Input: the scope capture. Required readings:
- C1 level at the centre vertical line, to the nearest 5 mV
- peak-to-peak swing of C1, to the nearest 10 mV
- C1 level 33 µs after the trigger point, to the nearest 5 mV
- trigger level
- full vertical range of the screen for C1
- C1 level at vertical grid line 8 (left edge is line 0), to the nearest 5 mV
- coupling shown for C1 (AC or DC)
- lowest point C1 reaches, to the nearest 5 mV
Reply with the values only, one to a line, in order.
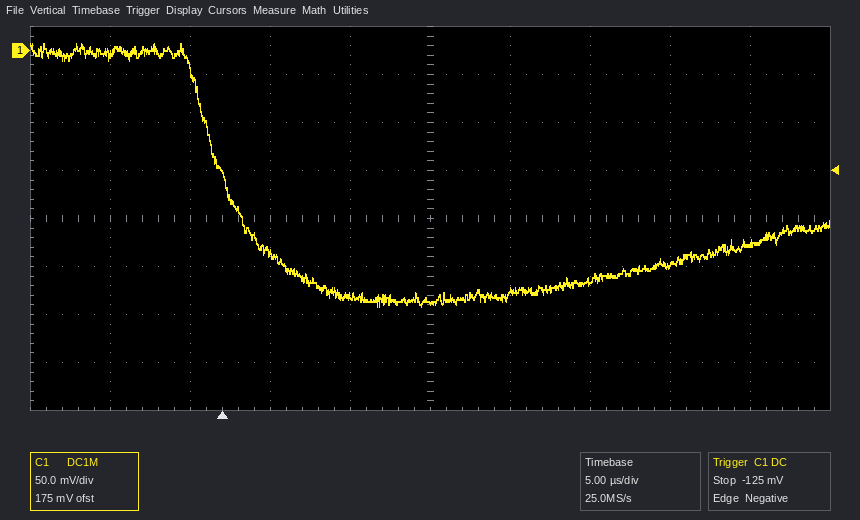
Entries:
-260 mV
270 mV
-200 mV
-125 mV
400 mV
-225 mV
DC
-265 mV
